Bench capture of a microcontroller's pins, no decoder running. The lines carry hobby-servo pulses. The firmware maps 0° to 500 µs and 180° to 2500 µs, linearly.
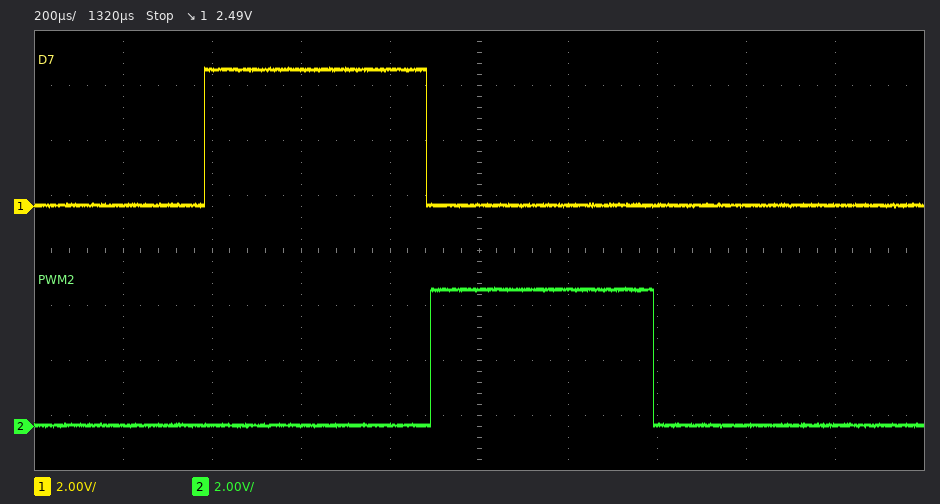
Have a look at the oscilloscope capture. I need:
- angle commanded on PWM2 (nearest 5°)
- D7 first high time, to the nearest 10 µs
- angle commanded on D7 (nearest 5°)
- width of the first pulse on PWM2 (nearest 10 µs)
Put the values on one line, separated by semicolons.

0°; 500 µs; 0°; 500 µs
